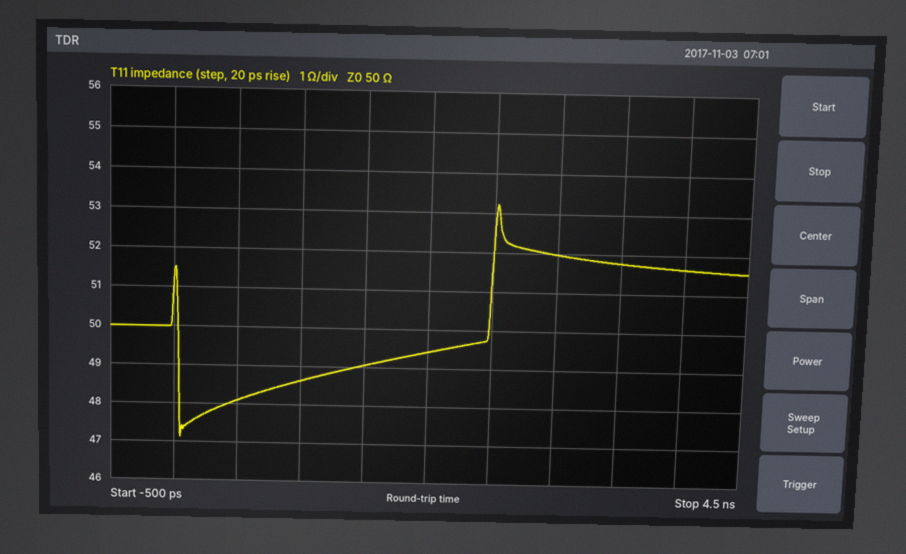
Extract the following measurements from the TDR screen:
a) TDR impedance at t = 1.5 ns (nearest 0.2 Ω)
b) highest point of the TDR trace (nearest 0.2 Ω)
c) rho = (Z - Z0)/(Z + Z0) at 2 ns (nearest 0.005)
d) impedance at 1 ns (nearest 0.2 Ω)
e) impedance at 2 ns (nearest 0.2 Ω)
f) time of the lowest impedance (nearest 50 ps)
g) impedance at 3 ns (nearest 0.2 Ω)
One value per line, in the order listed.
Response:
49.0 Ω
53.2 Ω
-0.005
48.6 Ω
49.4 Ω
50 ps
52.0 Ω
